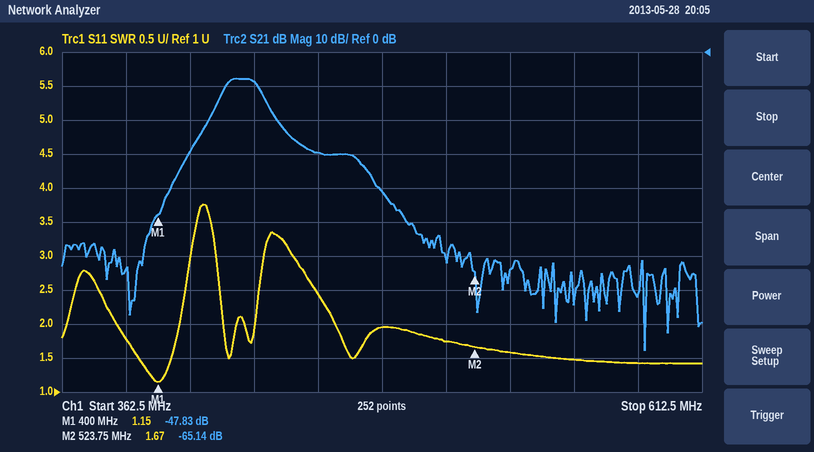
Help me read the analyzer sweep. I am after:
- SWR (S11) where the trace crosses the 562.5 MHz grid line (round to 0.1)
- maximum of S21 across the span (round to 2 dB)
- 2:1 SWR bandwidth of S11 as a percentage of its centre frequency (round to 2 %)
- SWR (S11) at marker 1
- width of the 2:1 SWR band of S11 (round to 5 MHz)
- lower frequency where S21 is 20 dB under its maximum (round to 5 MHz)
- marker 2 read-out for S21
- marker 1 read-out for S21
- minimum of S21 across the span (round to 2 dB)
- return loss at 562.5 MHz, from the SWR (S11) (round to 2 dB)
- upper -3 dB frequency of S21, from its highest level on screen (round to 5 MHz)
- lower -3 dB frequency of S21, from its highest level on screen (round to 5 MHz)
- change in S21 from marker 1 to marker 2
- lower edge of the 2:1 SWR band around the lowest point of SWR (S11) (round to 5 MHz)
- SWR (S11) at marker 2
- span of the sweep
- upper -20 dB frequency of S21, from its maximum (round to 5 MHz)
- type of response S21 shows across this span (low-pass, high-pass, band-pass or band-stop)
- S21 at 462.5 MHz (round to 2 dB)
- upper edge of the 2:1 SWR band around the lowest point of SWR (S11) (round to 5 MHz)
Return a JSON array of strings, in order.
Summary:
["1.5", "-8 dB", "6 %", "1.15", "25 MHz", "415 MHz", "-65.14 dB", "-47.83 dB", "-88 dB", "14 dB", "440 MHz", "425 MHz", "-17.31 dB", "385 MHz", "1.67", "250 MHz", "455 MHz", "band-pass", "-30 dB", "410 MHz"]
